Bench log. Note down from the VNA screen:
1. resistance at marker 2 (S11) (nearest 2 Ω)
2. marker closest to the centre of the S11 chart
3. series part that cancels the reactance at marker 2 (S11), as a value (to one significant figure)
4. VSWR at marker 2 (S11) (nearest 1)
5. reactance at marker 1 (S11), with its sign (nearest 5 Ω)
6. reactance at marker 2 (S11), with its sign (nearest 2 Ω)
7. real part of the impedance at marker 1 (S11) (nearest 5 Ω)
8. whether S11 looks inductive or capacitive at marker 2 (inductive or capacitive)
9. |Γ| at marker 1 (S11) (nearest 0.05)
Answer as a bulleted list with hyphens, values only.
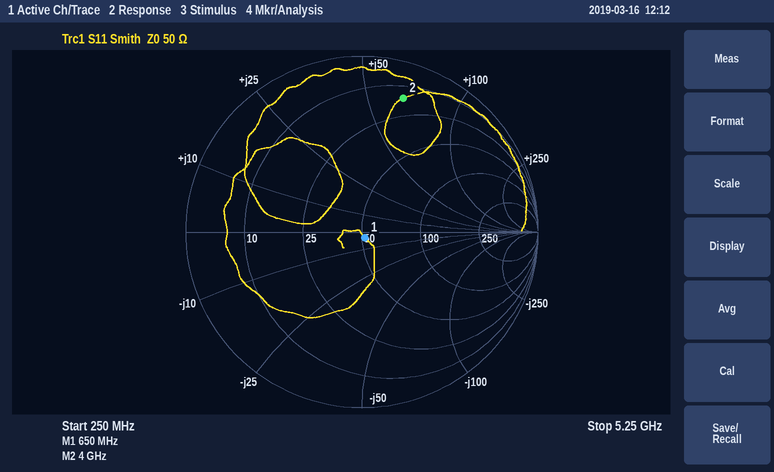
- 16 Ω
- marker 1
- 600 fF
- 9
- -5 Ω
- +66 Ω
- 50 Ω
- inductive
- 0.05
